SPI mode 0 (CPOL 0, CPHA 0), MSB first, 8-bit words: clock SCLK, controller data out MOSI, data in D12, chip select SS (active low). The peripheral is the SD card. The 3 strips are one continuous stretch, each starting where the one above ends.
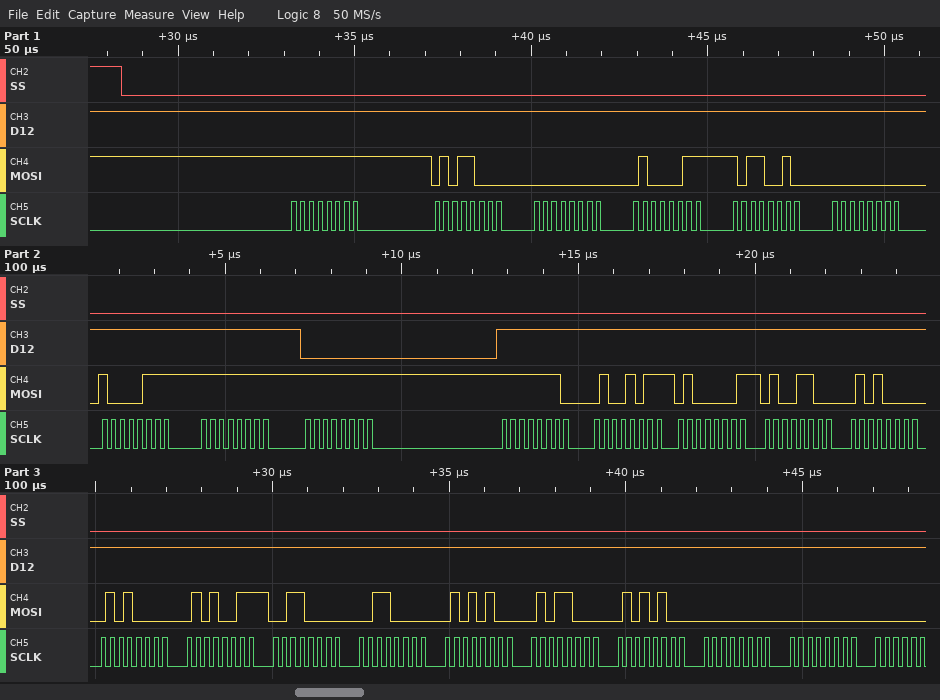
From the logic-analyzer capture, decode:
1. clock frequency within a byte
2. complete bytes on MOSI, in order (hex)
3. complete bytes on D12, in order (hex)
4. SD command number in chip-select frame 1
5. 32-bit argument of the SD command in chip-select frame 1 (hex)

4 MHz
FF 58 00 43 B2 00 87 FF FF FE 4B 41 4C 50 50 53 30 30 54 58 54 00 00
FF FF FF FF FF FF FF FF 00 FF FF FF FF FF FF FF FF FF FF FF FF FF FF
CMD24
0x0043B200
